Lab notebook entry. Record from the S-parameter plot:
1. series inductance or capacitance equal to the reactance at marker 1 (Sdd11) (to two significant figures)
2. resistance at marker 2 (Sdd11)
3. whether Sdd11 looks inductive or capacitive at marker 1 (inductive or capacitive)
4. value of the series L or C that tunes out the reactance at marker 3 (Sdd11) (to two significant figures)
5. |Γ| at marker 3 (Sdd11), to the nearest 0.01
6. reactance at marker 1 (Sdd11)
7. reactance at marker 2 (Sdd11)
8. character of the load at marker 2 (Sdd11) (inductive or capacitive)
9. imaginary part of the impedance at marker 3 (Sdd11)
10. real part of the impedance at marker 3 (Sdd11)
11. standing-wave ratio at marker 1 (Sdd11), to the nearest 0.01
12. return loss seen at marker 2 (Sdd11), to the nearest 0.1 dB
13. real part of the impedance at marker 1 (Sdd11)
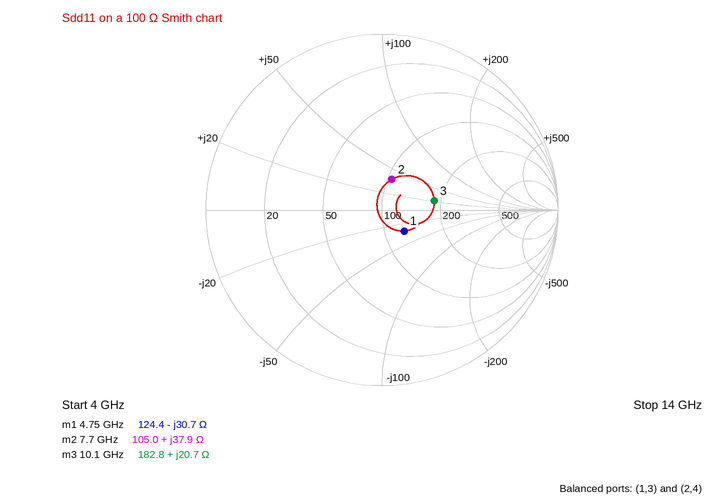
1.1 pF
105.0 Ω
capacitive
760 fF
0.30
-30.7 Ω
+37.9 Ω
inductive
+20.7 Ω
182.8 Ω
1.42
14.7 dB
124.4 Ω
